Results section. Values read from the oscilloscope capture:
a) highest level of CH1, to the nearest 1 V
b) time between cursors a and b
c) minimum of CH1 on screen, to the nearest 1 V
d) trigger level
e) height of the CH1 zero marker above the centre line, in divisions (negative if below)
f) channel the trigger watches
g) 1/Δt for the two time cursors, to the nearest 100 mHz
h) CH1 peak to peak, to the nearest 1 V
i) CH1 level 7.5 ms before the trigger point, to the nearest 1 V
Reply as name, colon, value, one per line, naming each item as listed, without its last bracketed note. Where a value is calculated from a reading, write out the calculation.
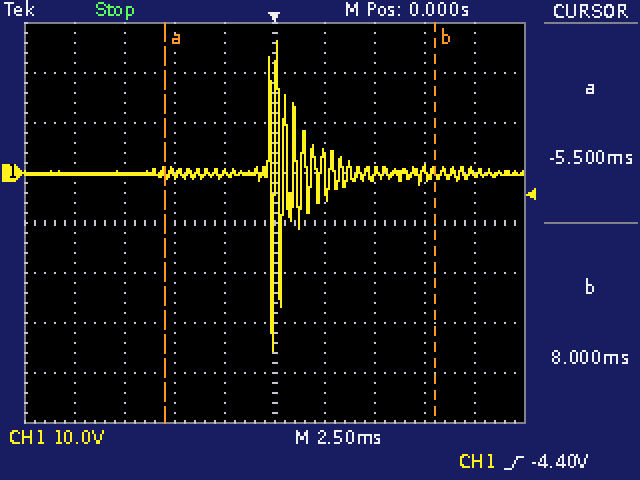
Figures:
highest level of CH1, to the nearest 1 V: 26 V
time between cursors a and b: 8 ms − (-5.5 ms) = 13.50 ms
minimum of CH1 on screen, to the nearest 1 V: -36 V
trigger level: -4.40 V
height of the CH1 zero marker above the centre line, in divisions: +1.0 div
channel the trigger watches: CH1
1/Δt for the two time cursors, to the nearest 100 mHz: 1 / 13.50 ms ≈ 74.1 Hz
CH1 peak to peak, to the nearest 1 V: 26 V − (-36 V) = 62 V
CH1 level 7.5 ms before the trigger point, to the nearest 1 V: 0 V
